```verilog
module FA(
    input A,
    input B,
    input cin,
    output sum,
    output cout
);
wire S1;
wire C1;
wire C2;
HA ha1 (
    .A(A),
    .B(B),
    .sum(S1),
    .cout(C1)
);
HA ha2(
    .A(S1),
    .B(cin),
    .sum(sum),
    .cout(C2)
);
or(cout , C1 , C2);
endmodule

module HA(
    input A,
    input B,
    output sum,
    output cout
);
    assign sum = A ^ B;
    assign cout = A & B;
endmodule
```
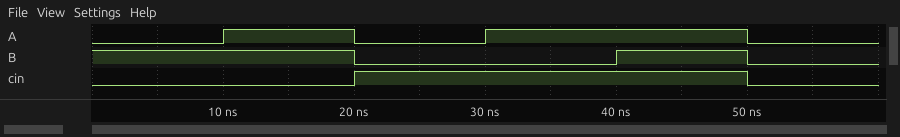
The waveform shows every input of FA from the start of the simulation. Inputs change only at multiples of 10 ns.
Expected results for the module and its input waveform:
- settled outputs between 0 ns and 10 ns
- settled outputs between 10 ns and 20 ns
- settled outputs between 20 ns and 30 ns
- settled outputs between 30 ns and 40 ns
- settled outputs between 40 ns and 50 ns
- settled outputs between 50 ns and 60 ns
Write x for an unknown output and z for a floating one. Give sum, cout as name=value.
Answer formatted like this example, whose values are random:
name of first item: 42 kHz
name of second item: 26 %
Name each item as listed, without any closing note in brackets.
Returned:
settled outputs between 0 ns and 10 ns: sum=1, cout=0
settled outputs between 10 ns and 20 ns: sum=0, cout=1
settled outputs between 20 ns and 30 ns: sum=1, cout=0
settled outputs between 30 ns and 40 ns: sum=0, cout=1
settled outputs between 40 ns and 50 ns: sum=1, cout=1
settled outputs between 50 ns and 60 ns: sum=0, cout=0
